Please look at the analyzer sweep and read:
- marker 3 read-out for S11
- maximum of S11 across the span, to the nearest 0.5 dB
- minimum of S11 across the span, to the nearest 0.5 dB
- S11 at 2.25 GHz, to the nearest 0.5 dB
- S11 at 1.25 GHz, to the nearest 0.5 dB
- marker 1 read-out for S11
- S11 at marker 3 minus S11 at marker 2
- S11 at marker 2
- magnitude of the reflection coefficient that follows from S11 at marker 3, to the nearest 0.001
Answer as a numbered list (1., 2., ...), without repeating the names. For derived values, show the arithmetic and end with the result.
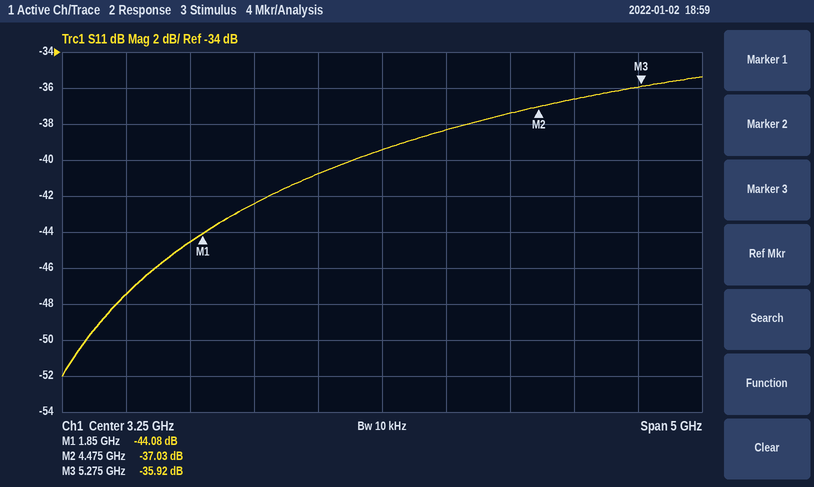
1. -35.92 dB
2. -35.5 dB
3. -52.0 dB
4. -42.5 dB
5. -47.5 dB
6. -44.08 dB
7. -35.92 − (-37.03) = 1.11 dB
8. -37.03 dB
9. 10^(-35.92/20) ≈ 0.016
